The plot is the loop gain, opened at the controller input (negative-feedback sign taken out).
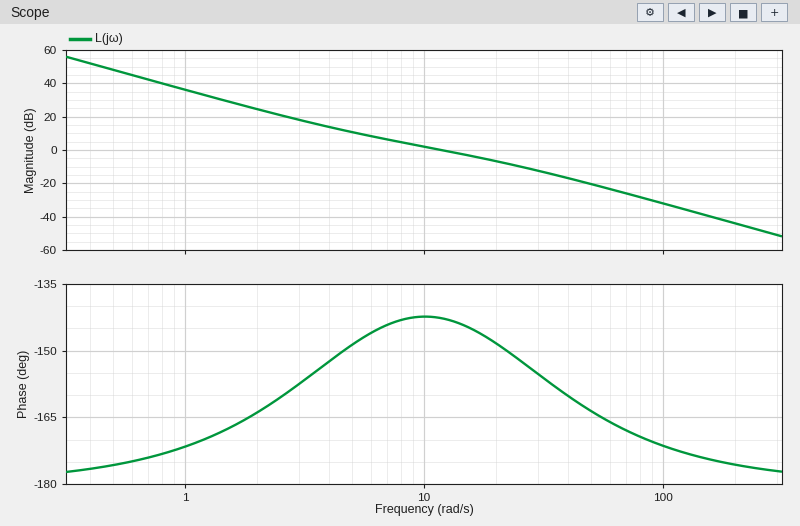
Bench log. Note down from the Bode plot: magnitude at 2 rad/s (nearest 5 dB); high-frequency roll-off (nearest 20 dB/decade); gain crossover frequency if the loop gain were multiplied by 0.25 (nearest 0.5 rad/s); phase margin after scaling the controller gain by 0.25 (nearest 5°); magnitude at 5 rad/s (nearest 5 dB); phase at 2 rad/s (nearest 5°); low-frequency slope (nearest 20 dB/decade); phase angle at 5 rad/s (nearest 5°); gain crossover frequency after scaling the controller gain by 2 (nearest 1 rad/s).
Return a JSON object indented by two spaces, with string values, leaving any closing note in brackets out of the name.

{
  "magnitude at 2 rad/s": "25 dB",
  "high-frequency roll-off": "-40 dB/decade",
  "gain crossover frequency if the loop gain were multiplied by 0.25": "4.5 rad/s",
  "phase margin after scaling the controller gain by 0.25": "30°",
  "magnitude at 5 rad/s": "10 dB",
  "phase at 2 rad/s": "-165°",
  "low-frequency slope": "-40 dB/decade",
  "phase angle at 5 rad/s": "-150°",
  "gain crossover frequency after scaling the controller gain by 2": "19 rad/s"
}
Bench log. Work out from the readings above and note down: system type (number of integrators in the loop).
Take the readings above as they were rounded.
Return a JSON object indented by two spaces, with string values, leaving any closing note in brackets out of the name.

{
  "system type": "2"
}
